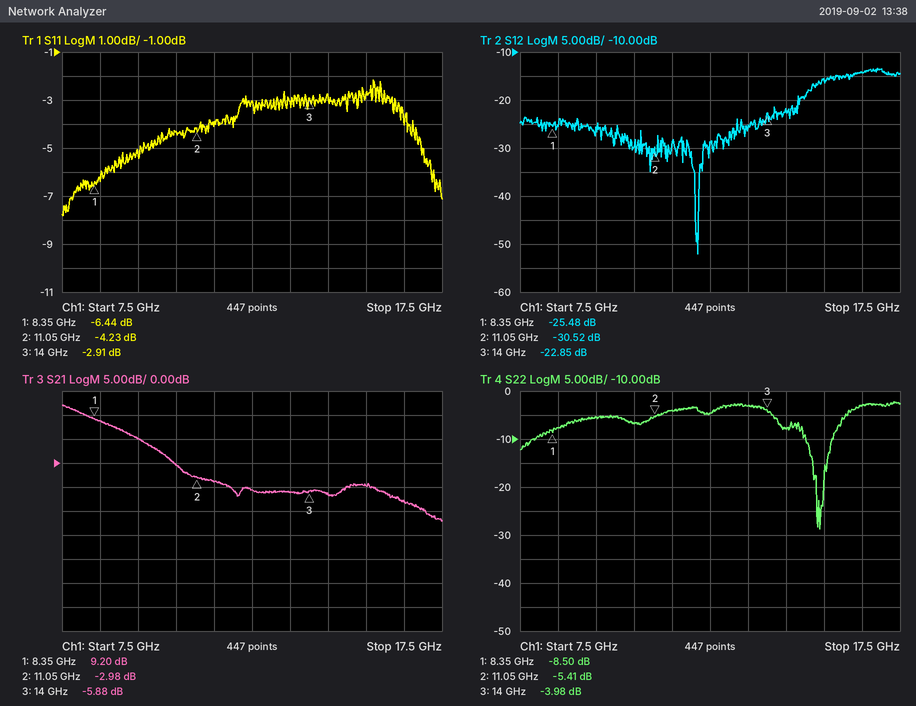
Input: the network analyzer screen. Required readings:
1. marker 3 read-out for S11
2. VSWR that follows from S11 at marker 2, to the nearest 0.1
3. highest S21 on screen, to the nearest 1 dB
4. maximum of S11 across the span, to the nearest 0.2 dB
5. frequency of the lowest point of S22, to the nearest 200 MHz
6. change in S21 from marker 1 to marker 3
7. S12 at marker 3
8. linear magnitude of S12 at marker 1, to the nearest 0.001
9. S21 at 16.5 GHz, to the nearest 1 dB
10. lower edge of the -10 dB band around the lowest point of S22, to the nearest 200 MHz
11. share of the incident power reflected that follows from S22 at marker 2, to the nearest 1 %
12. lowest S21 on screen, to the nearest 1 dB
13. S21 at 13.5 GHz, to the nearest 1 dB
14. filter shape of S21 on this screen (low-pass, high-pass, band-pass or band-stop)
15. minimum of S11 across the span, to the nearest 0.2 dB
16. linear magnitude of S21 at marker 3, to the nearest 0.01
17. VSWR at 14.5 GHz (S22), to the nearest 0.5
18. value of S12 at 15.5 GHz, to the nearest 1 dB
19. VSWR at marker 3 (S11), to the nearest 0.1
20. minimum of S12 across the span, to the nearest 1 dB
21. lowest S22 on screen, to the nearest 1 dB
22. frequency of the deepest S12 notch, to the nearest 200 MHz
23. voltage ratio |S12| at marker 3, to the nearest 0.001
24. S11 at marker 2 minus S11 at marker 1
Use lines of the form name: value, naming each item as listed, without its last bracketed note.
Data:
marker 3 read-out for S11: -2.91 dB
VSWR that follows from S11 at marker 2, to the nearest 0.1: 4.2
highest S21 on screen, to the nearest 1 dB: 12 dB
maximum of S11 across the span, to the nearest 0.2 dB: -2.2 dB
frequency of the lowest point of S22, to the nearest 200 MHz: 15.4 GHz
change in S21 from marker 1 to marker 3: -15.08 dB
S12 at marker 3: -22.85 dB
linear magnitude of S12 at marker 1, to the nearest 0.001: 0.053
S21 at 16.5 GHz, to the nearest 1 dB: -8 dB
lower edge of the -10 dB band around the lowest point of S22, to the nearest 200 MHz: 15.0 GHz
share of the incident power reflected that follows from S22 at marker 2, to the nearest 1 %: 29 %
lowest S21 on screen, to the nearest 1 dB: -12 dB
S21 at 13.5 GHz, to the nearest 1 dB: -6 dB
filter shape of S21 on this screen: low-pass
minimum of S11 across the span, to the nearest 0.2 dB: -7.8 dB
linear magnitude of S21 at marker 3, to the nearest 0.01: 0.51
VSWR at 14.5 GHz (S22), to the nearest 0.5: 2.5
value of S12 at 15.5 GHz, to the nearest 1 dB: -16 dB
VSWR at marker 3 (S11), to the nearest 0.1: 6.0
minimum of S12 across the span, to the nearest 1 dB: -52 dB
lowest S22 on screen, to the nearest 1 dB: -29 dB
frequency of the deepest S12 notch, to the nearest 200 MHz: 12.2 GHz
voltage ratio |S12| at marker 3, to the nearest 0.001: 0.072
S11 at marker 2 minus S11 at marker 1: 2.21 dB
